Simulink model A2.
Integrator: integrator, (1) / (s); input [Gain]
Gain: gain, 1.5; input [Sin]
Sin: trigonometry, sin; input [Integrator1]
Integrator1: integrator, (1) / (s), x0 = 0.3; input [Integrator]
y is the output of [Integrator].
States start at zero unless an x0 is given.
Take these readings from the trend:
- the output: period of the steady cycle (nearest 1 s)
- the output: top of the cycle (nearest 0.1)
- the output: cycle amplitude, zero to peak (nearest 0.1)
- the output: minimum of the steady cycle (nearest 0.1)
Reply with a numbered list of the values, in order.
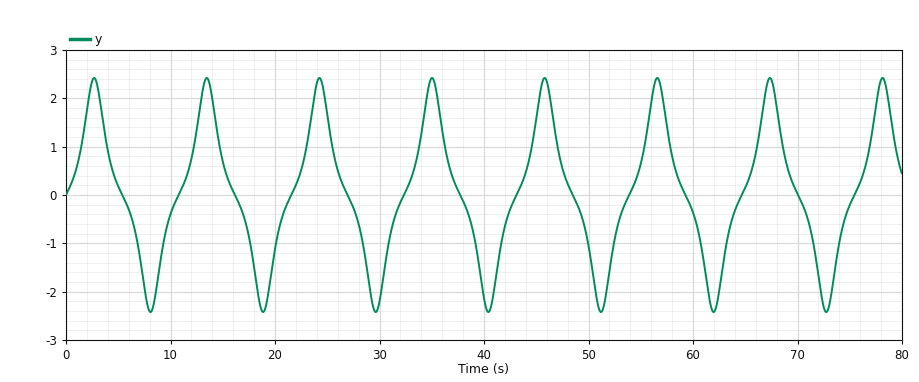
1. 11 s
2. 2.4
3. 2.4
4. -2.4
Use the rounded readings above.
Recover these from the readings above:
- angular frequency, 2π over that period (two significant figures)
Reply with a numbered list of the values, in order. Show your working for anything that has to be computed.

1. 2π / 11 = 0.57 rad/s
